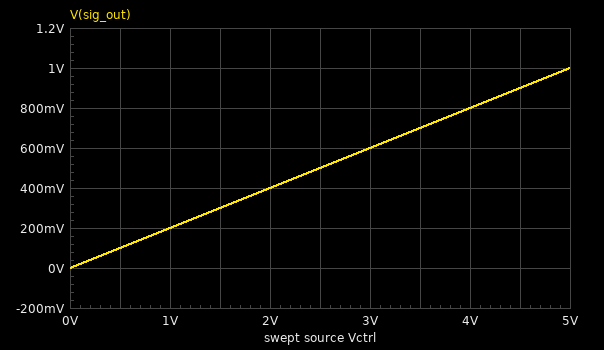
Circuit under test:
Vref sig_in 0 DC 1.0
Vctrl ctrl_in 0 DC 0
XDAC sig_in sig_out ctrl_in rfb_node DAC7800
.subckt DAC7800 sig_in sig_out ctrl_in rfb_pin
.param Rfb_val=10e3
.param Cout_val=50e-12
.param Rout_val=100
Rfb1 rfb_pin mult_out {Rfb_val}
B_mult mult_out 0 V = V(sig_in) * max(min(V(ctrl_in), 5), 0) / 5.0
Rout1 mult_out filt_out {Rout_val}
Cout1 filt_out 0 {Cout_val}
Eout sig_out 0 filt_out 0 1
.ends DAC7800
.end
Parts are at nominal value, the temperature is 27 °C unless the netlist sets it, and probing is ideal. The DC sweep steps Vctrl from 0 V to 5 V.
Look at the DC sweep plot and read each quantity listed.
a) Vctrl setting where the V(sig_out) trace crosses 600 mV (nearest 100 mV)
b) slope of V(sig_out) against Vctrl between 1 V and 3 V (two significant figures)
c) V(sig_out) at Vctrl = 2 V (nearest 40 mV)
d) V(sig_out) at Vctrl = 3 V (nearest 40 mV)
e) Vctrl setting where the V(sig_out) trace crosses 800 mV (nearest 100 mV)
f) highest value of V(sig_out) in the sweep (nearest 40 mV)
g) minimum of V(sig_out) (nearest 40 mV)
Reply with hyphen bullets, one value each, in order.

- 3.0 V
- 0.20 V/V
- 400 mV
- 600 mV
- 4.0 V
- 1.00 V
- 0 V
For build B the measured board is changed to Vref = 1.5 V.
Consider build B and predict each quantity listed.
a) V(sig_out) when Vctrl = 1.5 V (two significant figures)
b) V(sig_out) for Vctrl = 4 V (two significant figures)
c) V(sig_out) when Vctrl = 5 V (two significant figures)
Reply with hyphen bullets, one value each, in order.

- 450 mV
- 1.2 V
- 1.5 V
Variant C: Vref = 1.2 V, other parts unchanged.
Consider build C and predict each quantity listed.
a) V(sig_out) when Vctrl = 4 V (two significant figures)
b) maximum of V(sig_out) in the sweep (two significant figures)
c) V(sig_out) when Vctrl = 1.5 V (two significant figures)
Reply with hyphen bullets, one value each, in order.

- 960 mV
- 1.2 V
- 360 mV
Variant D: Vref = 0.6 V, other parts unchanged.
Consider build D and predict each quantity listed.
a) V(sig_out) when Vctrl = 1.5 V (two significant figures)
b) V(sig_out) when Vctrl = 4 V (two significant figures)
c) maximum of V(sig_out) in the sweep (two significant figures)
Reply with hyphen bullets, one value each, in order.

- 180 mV
- 480 mV
- 600 mV
